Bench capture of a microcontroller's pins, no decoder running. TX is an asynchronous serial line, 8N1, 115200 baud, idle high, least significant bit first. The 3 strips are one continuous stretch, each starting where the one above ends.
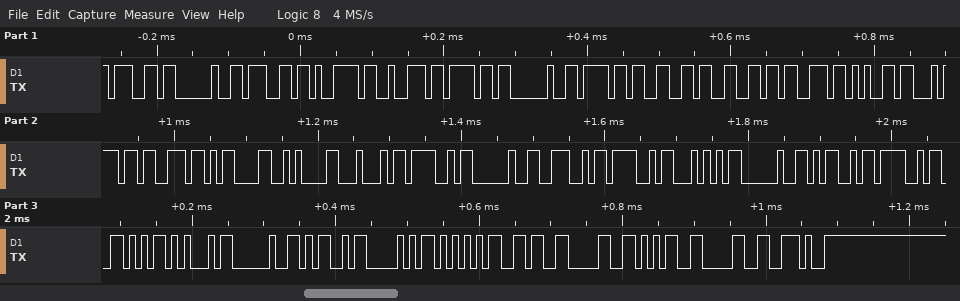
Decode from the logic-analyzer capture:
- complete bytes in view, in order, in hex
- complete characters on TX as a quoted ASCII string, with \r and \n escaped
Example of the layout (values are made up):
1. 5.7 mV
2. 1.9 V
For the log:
1. 67 20 67 79 72 6F 20 6F 66 66 73 65 74 73 0D 0A 44 4F 20 4E 4F 54 20 4D 4F 56 45 20 4D 50 55 36 30 35 30 2E
2. "g gyro offsets\r\nDO NOT MOVE MPU6050."
